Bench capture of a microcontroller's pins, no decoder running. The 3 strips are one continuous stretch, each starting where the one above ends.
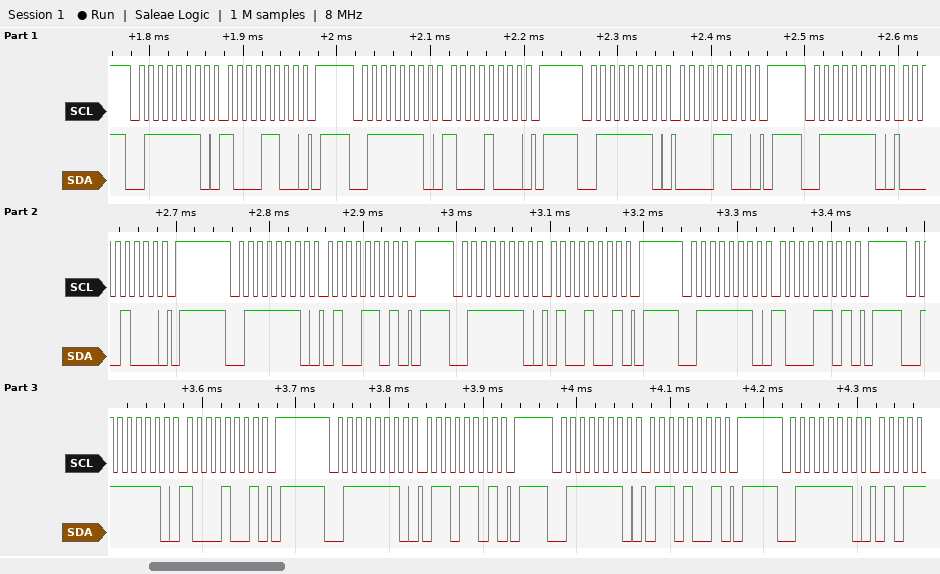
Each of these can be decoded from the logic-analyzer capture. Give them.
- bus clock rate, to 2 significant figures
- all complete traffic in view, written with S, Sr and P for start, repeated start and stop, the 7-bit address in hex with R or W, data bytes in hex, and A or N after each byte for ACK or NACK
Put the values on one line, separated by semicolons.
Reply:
100 kHz; S 3FW A 8C A P S 3FW A 88 A P S 3FW A 0C A P S 3FW A 08 A P S 3FW A 4D A P S 3FW A 49 A P S 3FW A 8D A P S 3FW A 89 A P S 3FW A 6D A P S 3FW A 69 A P S 3FW A
